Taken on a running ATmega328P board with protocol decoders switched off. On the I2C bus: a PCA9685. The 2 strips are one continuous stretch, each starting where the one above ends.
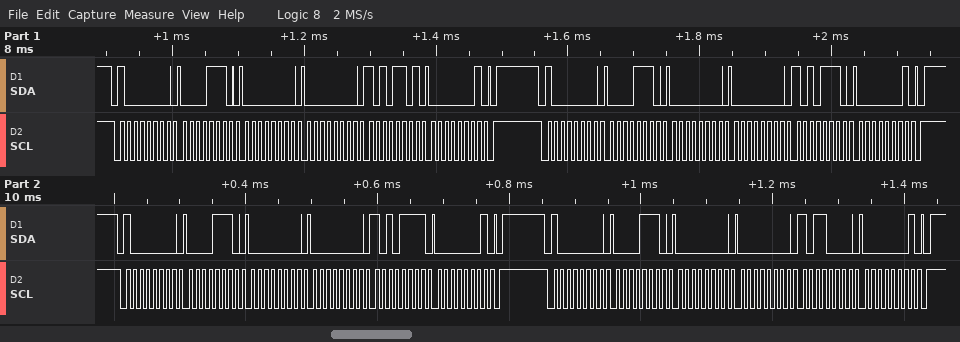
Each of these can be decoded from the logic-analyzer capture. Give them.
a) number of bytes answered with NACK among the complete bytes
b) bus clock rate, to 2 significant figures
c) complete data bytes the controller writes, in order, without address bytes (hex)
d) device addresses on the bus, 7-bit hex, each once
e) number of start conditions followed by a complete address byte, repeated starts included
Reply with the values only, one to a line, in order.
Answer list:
0
100 kHz
0E 00 00 AD 01 0E 00 00 AE 01 0E 00 00 AF 01 0E 00 00 B0 01
0x40
4
